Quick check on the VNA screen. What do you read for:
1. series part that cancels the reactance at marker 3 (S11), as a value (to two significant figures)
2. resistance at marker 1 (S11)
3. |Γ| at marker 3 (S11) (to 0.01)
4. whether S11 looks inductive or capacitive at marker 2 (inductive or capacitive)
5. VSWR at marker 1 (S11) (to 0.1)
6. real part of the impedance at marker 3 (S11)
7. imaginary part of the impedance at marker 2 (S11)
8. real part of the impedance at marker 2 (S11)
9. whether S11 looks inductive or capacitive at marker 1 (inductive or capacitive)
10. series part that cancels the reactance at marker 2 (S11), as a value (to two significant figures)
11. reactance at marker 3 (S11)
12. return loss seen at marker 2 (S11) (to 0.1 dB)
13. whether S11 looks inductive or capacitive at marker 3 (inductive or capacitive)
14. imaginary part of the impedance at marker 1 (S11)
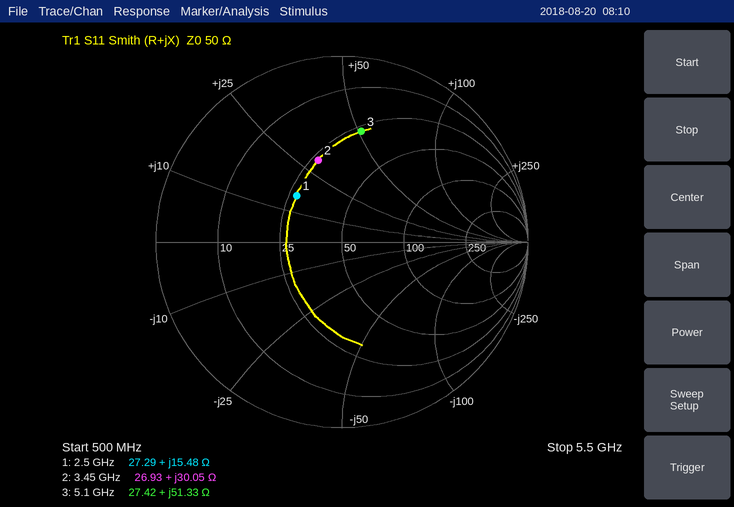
610 fF
27.29 Ω
0.60
inductive
2.1
27.42 Ω
+30.05 Ω
26.93 Ω
inductive
1.5 pF
+51.33 Ω
6.8 dB
inductive
+15.48 Ω
